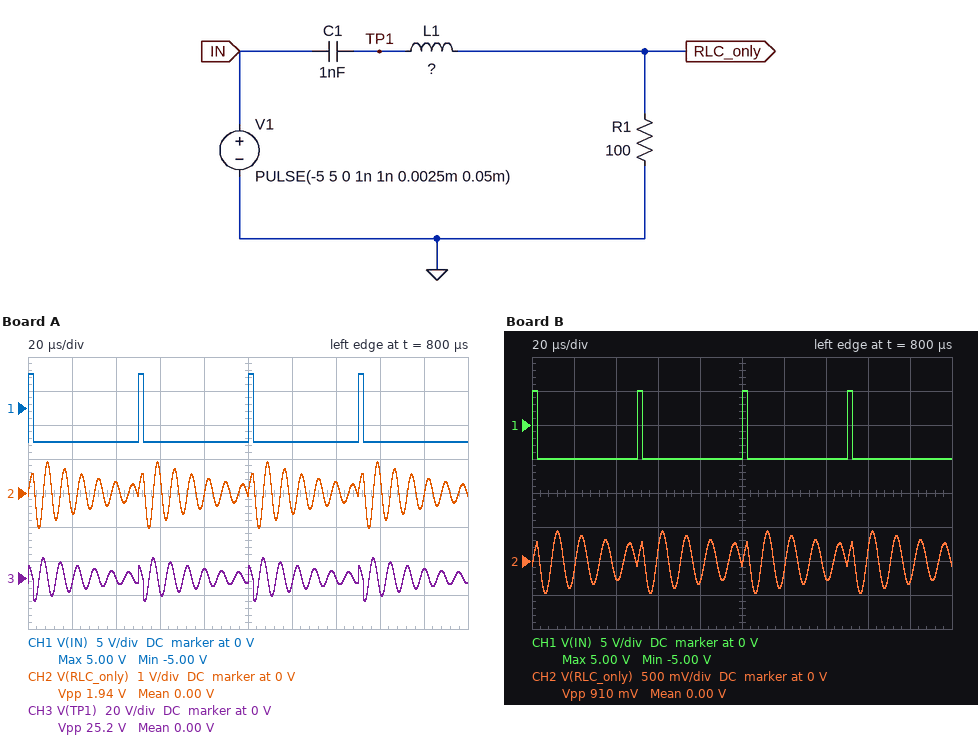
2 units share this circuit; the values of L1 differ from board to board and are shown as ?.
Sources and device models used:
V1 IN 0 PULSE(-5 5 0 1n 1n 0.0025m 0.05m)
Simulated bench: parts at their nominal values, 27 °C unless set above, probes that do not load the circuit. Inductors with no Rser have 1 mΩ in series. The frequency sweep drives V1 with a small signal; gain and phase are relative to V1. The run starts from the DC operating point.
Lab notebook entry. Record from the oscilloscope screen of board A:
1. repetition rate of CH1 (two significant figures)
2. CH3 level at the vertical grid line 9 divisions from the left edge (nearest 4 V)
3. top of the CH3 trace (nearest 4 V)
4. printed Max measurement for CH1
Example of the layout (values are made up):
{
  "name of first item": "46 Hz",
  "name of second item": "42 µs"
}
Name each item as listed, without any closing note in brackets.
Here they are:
{
  "repetition rate of CH1": "20 kHz",
  "CH3 level at the vertical grid line 9 divisions from the left edge": "4 V",
  "top of the CH3 trace": "12 V",
  "printed Max measurement for CH1": "5.00 V"
}
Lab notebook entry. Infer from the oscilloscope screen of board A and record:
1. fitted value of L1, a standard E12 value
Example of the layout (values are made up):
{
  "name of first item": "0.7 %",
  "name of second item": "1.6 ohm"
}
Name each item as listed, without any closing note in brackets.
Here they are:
{
  "fitted value of L1, a standard E12 value": "1.5 mH"
}
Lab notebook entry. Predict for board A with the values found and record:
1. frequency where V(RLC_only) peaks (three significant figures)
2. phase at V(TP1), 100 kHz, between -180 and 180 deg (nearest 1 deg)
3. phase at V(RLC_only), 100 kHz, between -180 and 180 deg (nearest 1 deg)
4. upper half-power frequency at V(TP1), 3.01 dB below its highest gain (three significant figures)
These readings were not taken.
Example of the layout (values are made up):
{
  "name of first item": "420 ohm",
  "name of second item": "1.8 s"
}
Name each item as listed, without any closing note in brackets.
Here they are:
{
  "frequency where V(RLC_only) peaks": "130 kHz",
  "phase at V(TP1), 100 kHz, between -180 and 180 deg": "165 deg",
  "phase at V(RLC_only), 100 kHz, between -180 and 180 deg": "81 deg",
  "upper half-power frequency at V(TP1), 3.01 dB below its highest gain": "136 kHz"
}
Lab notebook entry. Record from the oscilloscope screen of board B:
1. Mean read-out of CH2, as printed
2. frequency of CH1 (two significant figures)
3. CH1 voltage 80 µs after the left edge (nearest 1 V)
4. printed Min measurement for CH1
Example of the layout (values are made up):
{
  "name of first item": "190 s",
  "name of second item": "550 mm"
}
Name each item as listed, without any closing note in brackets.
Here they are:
{
  "Mean read-out of CH2, as printed": "0.00 V",
  "frequency of CH1": "20 kHz",
  "CH1 voltage 80 µs after the left edge": "-5 V",
  "printed Min measurement for CH1": "-5.00 V"
}
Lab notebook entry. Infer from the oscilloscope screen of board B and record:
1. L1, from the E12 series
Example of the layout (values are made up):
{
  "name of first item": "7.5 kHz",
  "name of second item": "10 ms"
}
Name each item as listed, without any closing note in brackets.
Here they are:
{
  "L1, from the E12 series": "3.3 mH"
}
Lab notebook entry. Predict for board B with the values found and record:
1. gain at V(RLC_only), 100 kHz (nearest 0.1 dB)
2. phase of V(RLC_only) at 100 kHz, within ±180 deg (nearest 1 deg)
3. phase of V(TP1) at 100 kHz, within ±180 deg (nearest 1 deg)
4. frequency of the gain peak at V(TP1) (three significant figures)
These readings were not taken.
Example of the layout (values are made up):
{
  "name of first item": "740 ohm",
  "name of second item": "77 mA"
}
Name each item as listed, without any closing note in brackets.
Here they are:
{
  "gain at V(RLC_only), 100 kHz": "-13.8 dB",
  "phase of V(RLC_only) at 100 kHz, within ±180 deg": "-78 deg",
  "phase of V(TP1) at 100 kHz, within ±180 deg": "9 deg",
  "frequency of the gain peak at V(TP1)": "87.7 kHz"
}
